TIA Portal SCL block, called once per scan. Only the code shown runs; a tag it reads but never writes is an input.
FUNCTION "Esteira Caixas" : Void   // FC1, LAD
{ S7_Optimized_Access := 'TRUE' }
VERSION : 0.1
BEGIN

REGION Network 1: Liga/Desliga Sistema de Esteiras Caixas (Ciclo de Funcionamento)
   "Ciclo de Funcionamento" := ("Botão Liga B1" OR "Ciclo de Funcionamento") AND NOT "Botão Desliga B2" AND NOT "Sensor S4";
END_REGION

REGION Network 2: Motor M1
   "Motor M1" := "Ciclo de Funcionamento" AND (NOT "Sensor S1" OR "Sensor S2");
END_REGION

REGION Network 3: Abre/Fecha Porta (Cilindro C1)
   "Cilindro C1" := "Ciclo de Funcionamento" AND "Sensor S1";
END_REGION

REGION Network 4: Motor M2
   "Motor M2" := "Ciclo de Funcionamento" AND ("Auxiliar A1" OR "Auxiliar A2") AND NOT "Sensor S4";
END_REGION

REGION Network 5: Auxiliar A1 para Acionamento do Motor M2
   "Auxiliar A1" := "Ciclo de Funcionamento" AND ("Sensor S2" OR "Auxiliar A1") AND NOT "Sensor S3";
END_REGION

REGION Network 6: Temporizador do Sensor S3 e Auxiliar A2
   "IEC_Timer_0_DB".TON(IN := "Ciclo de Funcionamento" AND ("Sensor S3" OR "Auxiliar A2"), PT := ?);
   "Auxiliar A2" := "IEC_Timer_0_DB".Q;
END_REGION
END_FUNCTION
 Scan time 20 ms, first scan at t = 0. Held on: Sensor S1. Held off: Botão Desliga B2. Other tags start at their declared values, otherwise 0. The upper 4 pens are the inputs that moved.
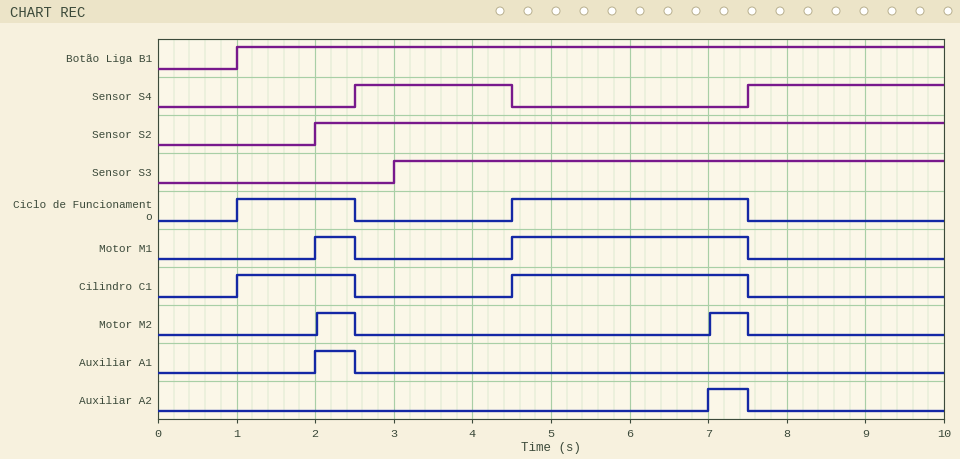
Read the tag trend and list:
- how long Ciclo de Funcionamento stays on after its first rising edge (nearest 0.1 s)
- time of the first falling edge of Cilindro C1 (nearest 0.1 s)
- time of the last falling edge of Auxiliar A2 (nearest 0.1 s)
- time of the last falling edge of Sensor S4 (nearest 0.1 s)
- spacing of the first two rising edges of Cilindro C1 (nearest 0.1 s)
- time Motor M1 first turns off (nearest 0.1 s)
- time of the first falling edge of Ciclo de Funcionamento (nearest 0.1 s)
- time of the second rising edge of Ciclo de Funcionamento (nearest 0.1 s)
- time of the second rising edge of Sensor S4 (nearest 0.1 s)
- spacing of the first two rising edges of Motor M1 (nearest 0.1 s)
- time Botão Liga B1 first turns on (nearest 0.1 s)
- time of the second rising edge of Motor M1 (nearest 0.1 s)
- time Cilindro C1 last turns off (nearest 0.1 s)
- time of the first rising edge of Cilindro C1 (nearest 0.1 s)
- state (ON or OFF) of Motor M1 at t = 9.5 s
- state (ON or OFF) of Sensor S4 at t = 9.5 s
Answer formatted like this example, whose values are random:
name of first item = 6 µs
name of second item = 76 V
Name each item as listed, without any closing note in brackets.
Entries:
how long Ciclo de Funcionamento stays on after its first rising edge = 1.5 s
time of the first falling edge of Cilindro C1 = 2.5 s
time of the last falling edge of Auxiliar A2 = 7.5 s
time of the last falling edge of Sensor S4 = 4.5 s
spacing of the first two rising edges of Cilindro C1 = 3.5 s
time Motor M1 first turns off = 2.5 s
time of the first falling edge of Ciclo de Funcionamento = 2.5 s
time of the second rising edge of Ciclo de Funcionamento = 4.5 s
time of the second rising edge of Sensor S4 = 7.5 s
spacing of the first two rising edges of Motor M1 = 2.5 s
time Botão Liga B1 first turns on = 1.0 s
time of the second rising edge of Motor M1 = 4.5 s
time Cilindro C1 last turns off = 7.5 s
time of the first rising edge of Cilindro C1 = 1.0 s
state (ON or OFF) of Motor M1 at t = 9.5 s = OFF
state (ON or OFF) of Sensor S4 at t = 9.5 s = ON
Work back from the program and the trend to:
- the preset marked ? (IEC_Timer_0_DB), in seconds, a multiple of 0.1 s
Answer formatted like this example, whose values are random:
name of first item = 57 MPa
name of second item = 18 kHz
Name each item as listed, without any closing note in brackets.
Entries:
the preset marked ? (IEC_Timer_0_DB), in seconds, a multiple of 0.1 s = 2.5 s
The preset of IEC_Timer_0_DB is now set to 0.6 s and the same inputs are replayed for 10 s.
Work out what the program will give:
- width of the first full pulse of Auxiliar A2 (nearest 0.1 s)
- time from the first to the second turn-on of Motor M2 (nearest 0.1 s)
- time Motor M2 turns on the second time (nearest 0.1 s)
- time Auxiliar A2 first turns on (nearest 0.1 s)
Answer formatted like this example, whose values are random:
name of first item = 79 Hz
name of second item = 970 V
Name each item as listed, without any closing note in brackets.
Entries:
width of the first full pulse of Auxiliar A2 = 2.4 s
time from the first to the second turn-on of Motor M2 = 3.1 s
time Motor M2 turns on the second time = 5.1 s
time Auxiliar A2 first turns on = 5.1 s
